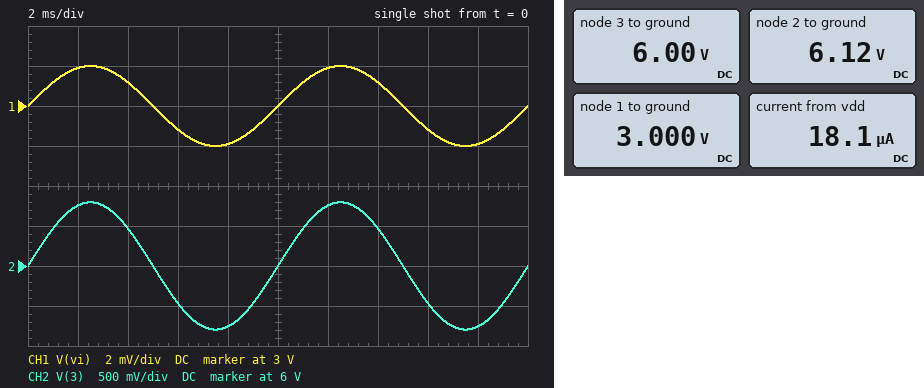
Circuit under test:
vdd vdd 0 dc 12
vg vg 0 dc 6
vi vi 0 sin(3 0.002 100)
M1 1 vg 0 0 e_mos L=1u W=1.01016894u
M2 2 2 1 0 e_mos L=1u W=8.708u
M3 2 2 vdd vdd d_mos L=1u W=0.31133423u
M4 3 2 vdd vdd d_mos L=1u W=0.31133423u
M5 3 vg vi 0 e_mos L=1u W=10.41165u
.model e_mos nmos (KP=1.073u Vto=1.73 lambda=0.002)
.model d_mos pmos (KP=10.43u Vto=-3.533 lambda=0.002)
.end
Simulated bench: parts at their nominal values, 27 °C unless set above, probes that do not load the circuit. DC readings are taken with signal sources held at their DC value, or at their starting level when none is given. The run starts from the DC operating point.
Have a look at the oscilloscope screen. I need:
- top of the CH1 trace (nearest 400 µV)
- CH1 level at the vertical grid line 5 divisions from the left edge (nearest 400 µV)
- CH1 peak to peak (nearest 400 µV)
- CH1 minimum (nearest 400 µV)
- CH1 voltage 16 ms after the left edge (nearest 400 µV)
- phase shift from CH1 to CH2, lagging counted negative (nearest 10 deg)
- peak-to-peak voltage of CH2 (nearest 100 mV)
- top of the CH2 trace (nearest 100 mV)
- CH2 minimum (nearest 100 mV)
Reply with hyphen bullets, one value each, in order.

- 3.0020 V
- 3.0000 V
- 4.0 mV
- 2.9980 V
- 2.9988 V
- 0 deg
- 1.6 V
- 6.8 V
- 5.2 V
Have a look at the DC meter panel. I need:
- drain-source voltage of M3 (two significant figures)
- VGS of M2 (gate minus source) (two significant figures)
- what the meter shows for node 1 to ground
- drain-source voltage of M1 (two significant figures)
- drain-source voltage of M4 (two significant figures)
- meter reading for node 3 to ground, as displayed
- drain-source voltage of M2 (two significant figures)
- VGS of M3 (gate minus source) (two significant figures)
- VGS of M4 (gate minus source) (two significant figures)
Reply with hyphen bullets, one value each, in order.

- -5.9 V
- 3.1 V
- 3.000 V
- 3.0 V
- -6.0 V
- 6.00 V
- 3.1 V
- -5.9 V
- -5.9 V
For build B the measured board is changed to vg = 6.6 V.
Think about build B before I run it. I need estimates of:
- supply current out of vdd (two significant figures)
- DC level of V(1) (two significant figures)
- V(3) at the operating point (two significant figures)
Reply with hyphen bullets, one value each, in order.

- 21 µA
- 2.7 V
- 3.6 V
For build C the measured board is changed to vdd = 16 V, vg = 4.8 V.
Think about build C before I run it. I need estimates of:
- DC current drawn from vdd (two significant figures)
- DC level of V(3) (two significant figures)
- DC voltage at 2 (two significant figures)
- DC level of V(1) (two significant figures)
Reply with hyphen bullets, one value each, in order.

- 5.2 µA
- 16 V
- 11 V
- 7.9 V
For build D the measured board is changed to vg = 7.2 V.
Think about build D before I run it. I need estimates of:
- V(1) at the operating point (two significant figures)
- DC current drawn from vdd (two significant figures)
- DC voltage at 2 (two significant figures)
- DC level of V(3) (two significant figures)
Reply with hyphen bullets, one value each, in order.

- 2.5 V
- 23 µA
- 5.8 V
- 3.5 V
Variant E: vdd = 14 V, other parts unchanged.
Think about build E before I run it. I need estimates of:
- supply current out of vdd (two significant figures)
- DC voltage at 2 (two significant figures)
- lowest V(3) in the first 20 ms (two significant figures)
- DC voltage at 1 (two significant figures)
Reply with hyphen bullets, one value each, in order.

- 19 µA
- 8.0 V
- 12 V
- 4.8 V
